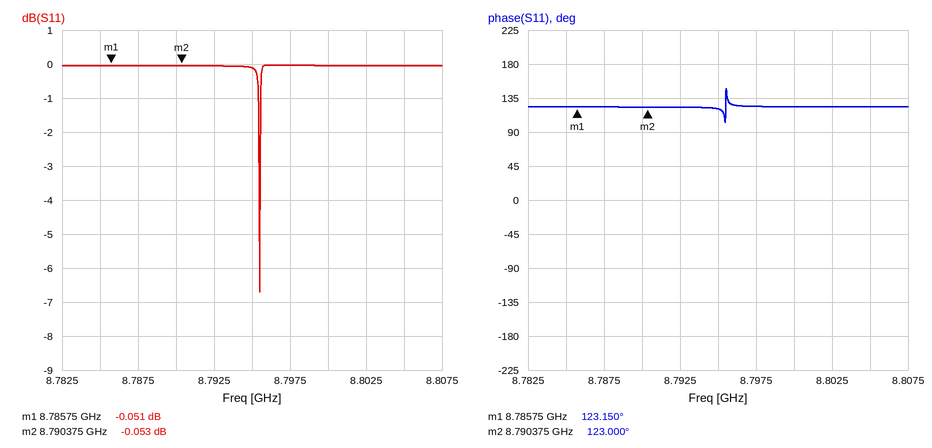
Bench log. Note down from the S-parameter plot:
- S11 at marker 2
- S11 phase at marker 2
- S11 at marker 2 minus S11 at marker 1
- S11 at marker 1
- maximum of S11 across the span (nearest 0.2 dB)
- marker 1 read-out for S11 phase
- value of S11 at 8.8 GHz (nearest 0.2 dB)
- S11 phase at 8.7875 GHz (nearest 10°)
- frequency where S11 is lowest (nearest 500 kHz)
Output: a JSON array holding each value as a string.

["-0.053 dB", "123.000°", "-0.002 dB", "-0.051 dB", "0.0 dB", "123.150°", "0.0 dB", "120°", "8.7955 GHz"]
